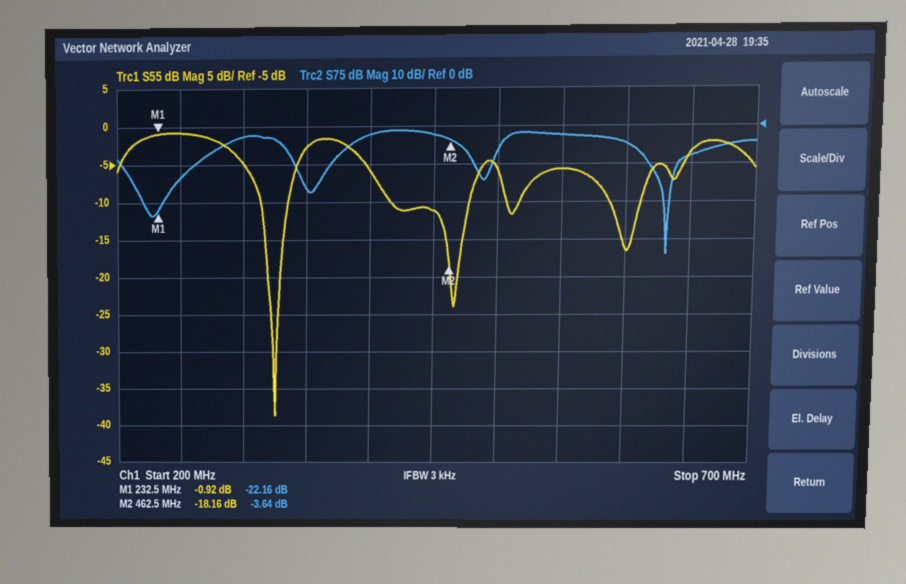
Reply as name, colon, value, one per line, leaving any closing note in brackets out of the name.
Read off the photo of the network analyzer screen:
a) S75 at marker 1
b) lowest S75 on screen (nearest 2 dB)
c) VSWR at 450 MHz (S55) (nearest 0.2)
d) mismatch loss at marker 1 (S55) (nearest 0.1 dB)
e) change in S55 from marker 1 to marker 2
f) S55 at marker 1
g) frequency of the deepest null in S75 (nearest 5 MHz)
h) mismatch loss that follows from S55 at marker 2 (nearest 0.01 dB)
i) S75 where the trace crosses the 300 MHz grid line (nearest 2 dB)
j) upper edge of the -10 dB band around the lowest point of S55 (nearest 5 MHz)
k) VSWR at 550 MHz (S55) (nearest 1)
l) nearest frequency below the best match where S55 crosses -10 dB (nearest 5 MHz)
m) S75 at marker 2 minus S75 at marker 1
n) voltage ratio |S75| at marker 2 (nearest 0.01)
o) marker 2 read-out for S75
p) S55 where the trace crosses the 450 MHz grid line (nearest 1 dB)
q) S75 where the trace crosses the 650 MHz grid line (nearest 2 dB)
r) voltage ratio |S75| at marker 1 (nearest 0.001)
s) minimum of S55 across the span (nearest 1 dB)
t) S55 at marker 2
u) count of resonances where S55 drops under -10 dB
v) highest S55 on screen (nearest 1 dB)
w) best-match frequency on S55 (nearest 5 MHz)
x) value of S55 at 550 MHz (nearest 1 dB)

S75 at marker 1: -22.16 dB
lowest S75 on screen: -34 dB
VSWR at 450 MHz (S55): 1.8
mismatch loss at marker 1 (S55): 7.2 dB
change in S55 from marker 1 to marker 2: -17.24 dB
S55 at marker 1: -0.92 dB
frequency of the deepest null in S75: 630 MHz
mismatch loss that follows from S55 at marker 2: 0.07 dB
S75 where the trace crosses the 300 MHz grid line: -2 dB
upper edge of the -10 dB band around the lowest point of S55: 335 MHz
VSWR at 550 MHz (S55): 3
nearest frequency below the best match where S55 crosses -10 dB: 315 MHz
S75 at marker 2 minus S75 at marker 1: 18.52 dB
voltage ratio |S75| at marker 2: 0.66
marker 2 read-out for S75: -3.64 dB
S55 where the trace crosses the 450 MHz grid line: -11 dB
S75 where the trace crosses the 650 MHz grid line: -8 dB
voltage ratio |S75| at marker 1: 0.078
minimum of S55 across the span: -39 dB
S55 at marker 2: -18.16 dB
count of resonances where S55 drops under -10 dB: 4
highest S55 on screen: -1 dB
best-match frequency on S55: 325 MHz
value of S55 at 550 MHz: -6 dB
